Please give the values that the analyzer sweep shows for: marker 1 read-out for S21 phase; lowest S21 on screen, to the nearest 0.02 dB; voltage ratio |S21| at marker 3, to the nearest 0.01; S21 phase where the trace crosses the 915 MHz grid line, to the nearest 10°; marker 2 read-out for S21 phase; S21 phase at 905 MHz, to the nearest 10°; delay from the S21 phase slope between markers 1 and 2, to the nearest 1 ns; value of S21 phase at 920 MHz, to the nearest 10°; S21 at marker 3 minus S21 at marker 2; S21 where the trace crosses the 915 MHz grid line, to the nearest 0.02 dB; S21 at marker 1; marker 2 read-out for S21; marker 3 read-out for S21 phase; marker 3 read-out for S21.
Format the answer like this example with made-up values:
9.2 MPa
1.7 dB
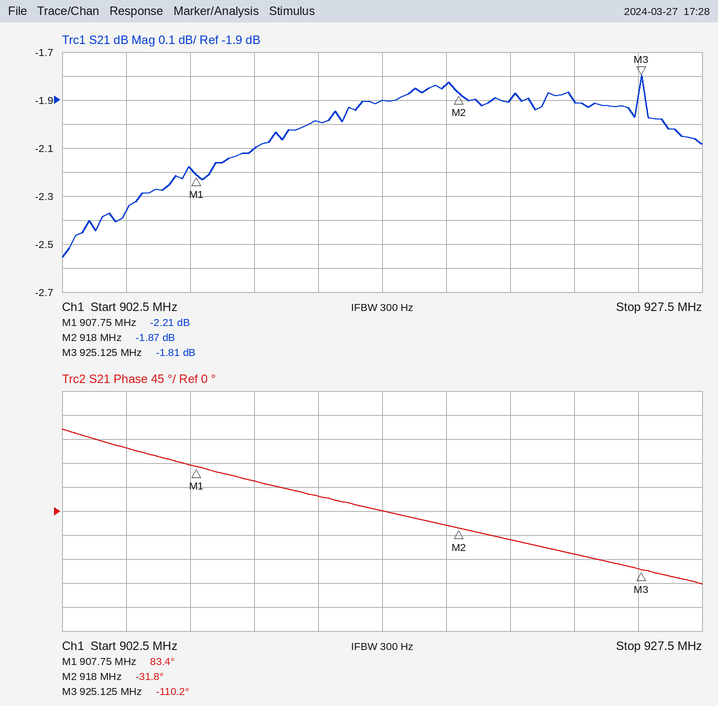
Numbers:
83.4°
-2.56 dB
0.81
0°
-31.8°
120°
31 ns
-50°
0.06 dB
-1.90 dB
-2.21 dB
-1.87 dB
-110.2°
-1.81 dB
